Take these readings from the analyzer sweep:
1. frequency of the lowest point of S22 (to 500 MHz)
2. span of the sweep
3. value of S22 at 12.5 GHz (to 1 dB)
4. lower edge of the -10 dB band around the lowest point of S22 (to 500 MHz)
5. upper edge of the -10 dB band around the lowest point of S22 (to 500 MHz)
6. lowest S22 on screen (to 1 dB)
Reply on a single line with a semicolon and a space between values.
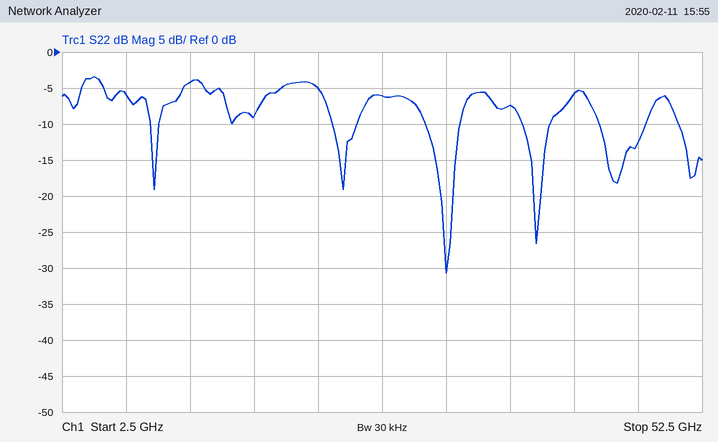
32.5 GHz; 50 GHz; -4 dB; 31.0 GHz; 33.5 GHz; -31 dB
